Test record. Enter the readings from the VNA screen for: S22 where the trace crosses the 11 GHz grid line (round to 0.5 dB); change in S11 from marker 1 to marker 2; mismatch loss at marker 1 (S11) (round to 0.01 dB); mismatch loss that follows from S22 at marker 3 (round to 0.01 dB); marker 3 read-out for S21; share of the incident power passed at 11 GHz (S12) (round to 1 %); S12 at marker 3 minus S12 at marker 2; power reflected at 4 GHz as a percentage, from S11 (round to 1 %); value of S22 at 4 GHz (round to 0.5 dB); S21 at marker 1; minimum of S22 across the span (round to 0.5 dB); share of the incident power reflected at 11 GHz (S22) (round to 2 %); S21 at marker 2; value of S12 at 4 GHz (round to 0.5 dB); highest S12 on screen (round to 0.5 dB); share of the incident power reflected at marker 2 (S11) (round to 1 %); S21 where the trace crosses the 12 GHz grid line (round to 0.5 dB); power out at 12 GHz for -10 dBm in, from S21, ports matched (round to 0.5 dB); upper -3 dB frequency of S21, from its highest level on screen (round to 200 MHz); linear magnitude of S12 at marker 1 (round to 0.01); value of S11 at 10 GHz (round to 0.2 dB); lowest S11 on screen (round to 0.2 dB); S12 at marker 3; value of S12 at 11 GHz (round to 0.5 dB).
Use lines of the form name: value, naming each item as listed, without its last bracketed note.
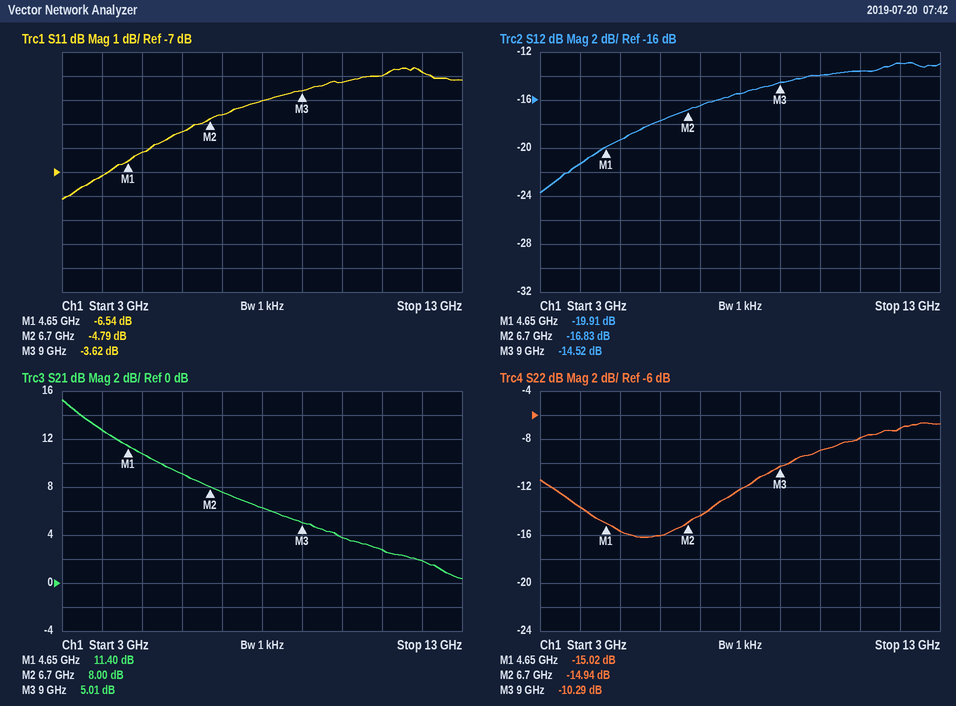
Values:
S22 where the trace crosses the 11 GHz grid line: -8.0 dB
change in S11 from marker 1 to marker 2: 1.75 dB
mismatch loss at marker 1 (S11): 1.09 dB
mismatch loss that follows from S22 at marker 3: 0.43 dB
marker 3 read-out for S21: 5.01 dB
share of the incident power passed at 11 GHz (S12): 4 %
S12 at marker 3 minus S12 at marker 2: 2.31 dB
power reflected at 4 GHz as a percentage, from S11: 19 %
value of S22 at 4 GHz: -13.5 dB
S21 at marker 1: 11.40 dB
minimum of S22 across the span: -16.0 dB
share of the incident power reflected at 11 GHz (S22): 16 %
S21 at marker 2: 8.00 dB
value of S12 at 4 GHz: -21.5 dB
highest S12 on screen: -13.0 dB
share of the incident power reflected at marker 2 (S11): 33 %
S21 where the trace crosses the 12 GHz grid line: 2.0 dB
power out at 12 GHz for -10 dBm in, from S21, ports matched: -8.0 dBm
upper -3 dB frequency of S21, from its highest level on screen: 4.2 GHz
linear magnitude of S12 at marker 1: 0.10
value of S11 at 10 GHz: -3.2 dB
lowest S11 on screen: -8.2 dB
S12 at marker 3: -14.52 dB
value of S12 at 11 GHz: -13.5 dB
